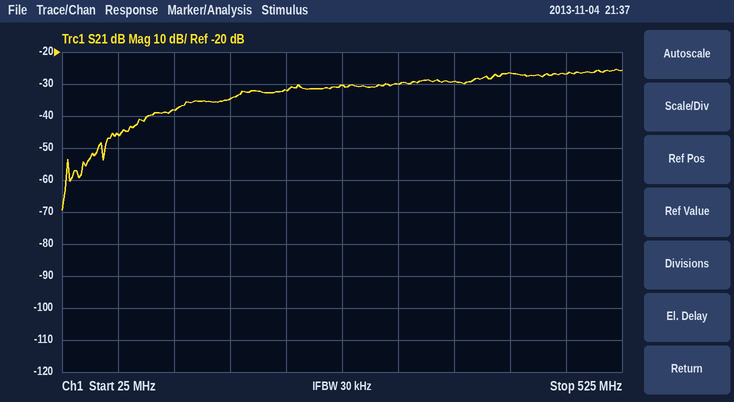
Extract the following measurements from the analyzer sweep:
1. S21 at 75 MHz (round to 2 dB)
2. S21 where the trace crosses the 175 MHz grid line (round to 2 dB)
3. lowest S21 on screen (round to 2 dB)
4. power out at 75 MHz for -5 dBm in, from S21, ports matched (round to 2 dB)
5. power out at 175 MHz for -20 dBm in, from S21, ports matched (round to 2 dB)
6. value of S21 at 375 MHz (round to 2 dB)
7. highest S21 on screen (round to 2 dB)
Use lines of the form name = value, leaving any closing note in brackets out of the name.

S21 at 75 MHz = -46 dB
S21 where the trace crosses the 175 MHz grid line = -34 dB
lowest S21 on screen = -70 dB
power out at 75 MHz for -5 dBm in, from S21, ports matched = -50 dBm
power out at 175 MHz for -20 dBm in, from S21, ports matched = -54 dBm
value of S21 at 375 MHz = -30 dB
highest S21 on screen = -26 dB
